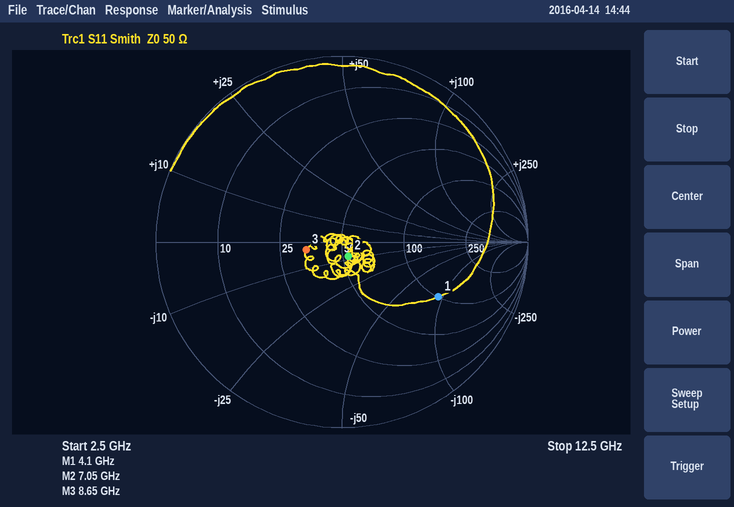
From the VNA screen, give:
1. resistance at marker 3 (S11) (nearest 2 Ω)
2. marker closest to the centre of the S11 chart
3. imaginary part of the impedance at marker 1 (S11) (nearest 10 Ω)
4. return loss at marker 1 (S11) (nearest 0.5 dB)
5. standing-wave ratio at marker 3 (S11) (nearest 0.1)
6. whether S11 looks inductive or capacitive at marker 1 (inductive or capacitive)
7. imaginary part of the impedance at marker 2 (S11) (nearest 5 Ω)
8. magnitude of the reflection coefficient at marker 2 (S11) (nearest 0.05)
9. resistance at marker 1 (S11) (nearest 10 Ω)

34 Ω
marker 2
-90 Ω
4.5 dB
1.5
capacitive
-10 Ω
0.10
100 Ω
